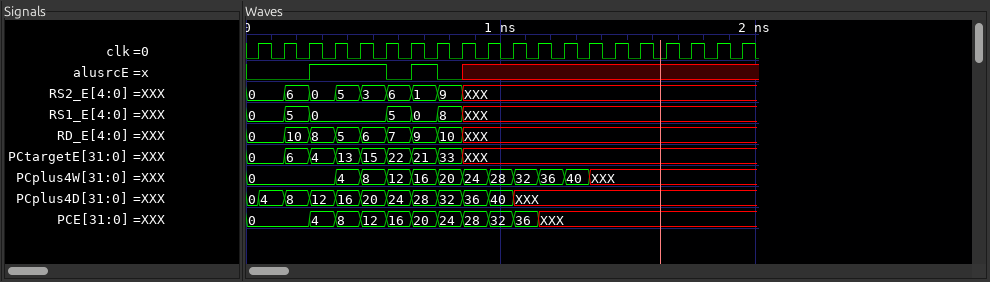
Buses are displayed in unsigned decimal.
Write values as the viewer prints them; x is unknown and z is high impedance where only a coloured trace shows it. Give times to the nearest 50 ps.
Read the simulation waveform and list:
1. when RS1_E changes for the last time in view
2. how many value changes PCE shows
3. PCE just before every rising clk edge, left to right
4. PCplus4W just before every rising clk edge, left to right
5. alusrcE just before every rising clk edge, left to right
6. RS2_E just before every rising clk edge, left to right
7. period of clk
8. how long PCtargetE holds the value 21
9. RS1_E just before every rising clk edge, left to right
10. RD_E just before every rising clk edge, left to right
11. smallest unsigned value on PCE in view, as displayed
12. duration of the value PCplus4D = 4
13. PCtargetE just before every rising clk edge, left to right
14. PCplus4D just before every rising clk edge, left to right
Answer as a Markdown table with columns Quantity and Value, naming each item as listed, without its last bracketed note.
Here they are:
| Quantity | Value |
|---|---|
| when RS1_E changes for the last time in view | 850 ps |
| how many value changes PCE shows | 10 |
| PCE just before every rising clk edge, left to right | 0, 0, 0, 4, 8, 12, 16, 20, 24, 28, 32, 36, XXX, XXX, XXX, XXX, XXX, XXX, XXX, XXX |
| PCplus4W just before every rising clk edge, left to right | 0, 0, 0, 0, 4, 8, 12, 16, 20, 24, 28, 32, 36, 40, XXX, XXX, XXX, XXX, XXX, XXX |
| alusrcE just before every rising clk edge, left to right | 0 0 0 1 1 1 0 1 0 x x x x x x x x x x x |
| RS2_E just before every rising clk edge, left to right | 0, 0, 6, 0, 5, 3, 6, 1, 9, XXX, XXX, XXX, XXX, XXX, XXX, XXX, XXX, XXX, XXX, XXX |
| period of clk | 100 ps |
| how long PCtargetE holds the value 21 | 100 ps |
| RS1_E just before every rising clk edge, left to right | 0, 0, 5, 0, 0, 0, 5, 0, 8, XXX, XXX, XXX, XXX, XXX, XXX, XXX, XXX, XXX, XXX, XXX |
| RD_E just before every rising clk edge, left to right | 0, 0, 10, 8, 5, 6, 7, 9, 10, XXX, XXX, XXX, XXX, XXX, XXX, XXX, XXX, XXX, XXX, XXX |
| smallest unsigned value on PCE in view, as displayed | 0 |
| duration of the value PCplus4D = 4 | 100 ps |
| PCtargetE just before every rising clk edge, left to right | 0, 0, 6, 4, 13, 15, 22, 21, 33, XXX, XXX, XXX, XXX, XXX, XXX, XXX, XXX, XXX, XXX, XXX |
| PCplus4D just before every rising clk edge, left to right | 0, 4, 8, 12, 16, 20, 24, 28, 32, 36, 40, XXX, XXX, XXX, XXX, XXX, XXX, XXX, XXX, XXX |
